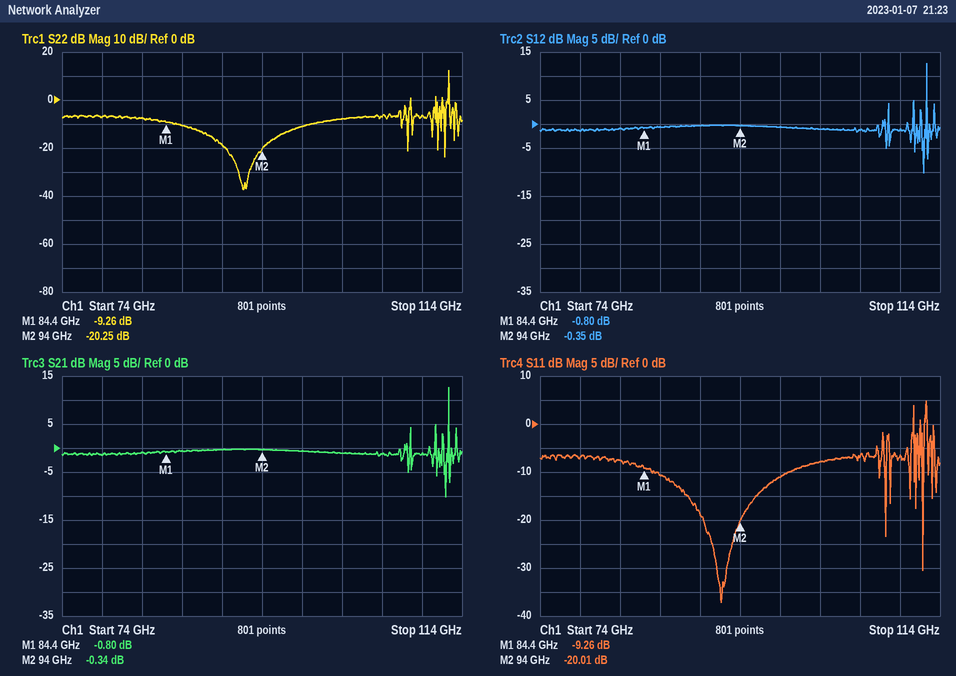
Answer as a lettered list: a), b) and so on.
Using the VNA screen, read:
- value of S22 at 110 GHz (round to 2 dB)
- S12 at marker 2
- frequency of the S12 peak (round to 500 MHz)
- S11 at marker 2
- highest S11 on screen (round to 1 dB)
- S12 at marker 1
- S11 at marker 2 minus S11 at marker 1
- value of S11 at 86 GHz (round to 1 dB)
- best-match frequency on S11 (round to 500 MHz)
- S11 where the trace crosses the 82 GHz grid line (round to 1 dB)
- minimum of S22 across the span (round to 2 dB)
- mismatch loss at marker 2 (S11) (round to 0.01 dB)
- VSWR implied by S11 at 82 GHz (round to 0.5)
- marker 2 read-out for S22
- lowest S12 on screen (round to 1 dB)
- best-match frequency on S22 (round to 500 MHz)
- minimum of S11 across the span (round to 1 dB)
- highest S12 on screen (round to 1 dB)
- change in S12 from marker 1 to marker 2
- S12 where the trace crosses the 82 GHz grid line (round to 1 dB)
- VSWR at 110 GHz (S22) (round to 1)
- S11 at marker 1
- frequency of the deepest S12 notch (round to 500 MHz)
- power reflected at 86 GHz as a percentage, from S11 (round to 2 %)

a) -6 dB
b) -0.35 dB
c) 112.5 GHz
d) -20.01 dB
e) 5 dB
f) -0.80 dB
g) -10.75 dB
h) -11 dB
i) 92.0 GHz
j) -8 dB
k) -38 dB
l) 0.04 dB
m) 2.5
n) -20.25 dB
o) -10 dB
p) 92.0 GHz
q) -37 dB
r) 13 dB
s) 0.45 dB
t) -1 dB
u) 3
v) -9.26 dB
w) 112.5 GHz
x) 8 %
